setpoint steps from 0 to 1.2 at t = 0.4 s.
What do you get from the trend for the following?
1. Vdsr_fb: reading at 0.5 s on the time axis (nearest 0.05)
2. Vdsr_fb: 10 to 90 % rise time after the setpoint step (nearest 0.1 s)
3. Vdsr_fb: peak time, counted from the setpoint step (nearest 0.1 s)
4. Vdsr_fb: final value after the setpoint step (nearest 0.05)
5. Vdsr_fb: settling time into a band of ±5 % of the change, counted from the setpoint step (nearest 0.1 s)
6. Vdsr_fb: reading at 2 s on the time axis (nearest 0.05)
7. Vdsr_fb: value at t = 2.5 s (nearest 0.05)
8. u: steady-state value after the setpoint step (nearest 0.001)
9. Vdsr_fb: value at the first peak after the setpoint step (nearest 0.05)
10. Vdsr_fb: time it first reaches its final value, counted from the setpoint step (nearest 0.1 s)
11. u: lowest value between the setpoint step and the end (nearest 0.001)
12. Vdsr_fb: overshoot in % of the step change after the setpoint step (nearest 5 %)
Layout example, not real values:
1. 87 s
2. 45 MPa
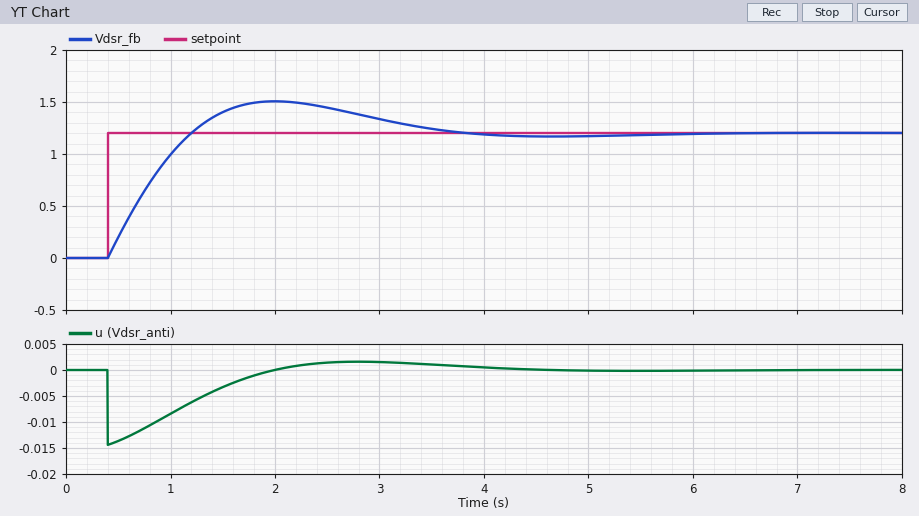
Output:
1. 0.20
2. 0.6 s
3. 1.6 s
4. 1.20
5. 3.0 s
6. 1.50
7. 1.45
8. 0.000
9. 1.50
10. 0.8 s
11. -0.014
12. 25 %
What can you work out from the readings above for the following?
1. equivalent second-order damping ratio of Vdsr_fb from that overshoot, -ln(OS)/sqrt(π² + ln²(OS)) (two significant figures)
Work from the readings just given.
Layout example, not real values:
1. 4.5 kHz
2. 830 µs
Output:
1. 0.40
